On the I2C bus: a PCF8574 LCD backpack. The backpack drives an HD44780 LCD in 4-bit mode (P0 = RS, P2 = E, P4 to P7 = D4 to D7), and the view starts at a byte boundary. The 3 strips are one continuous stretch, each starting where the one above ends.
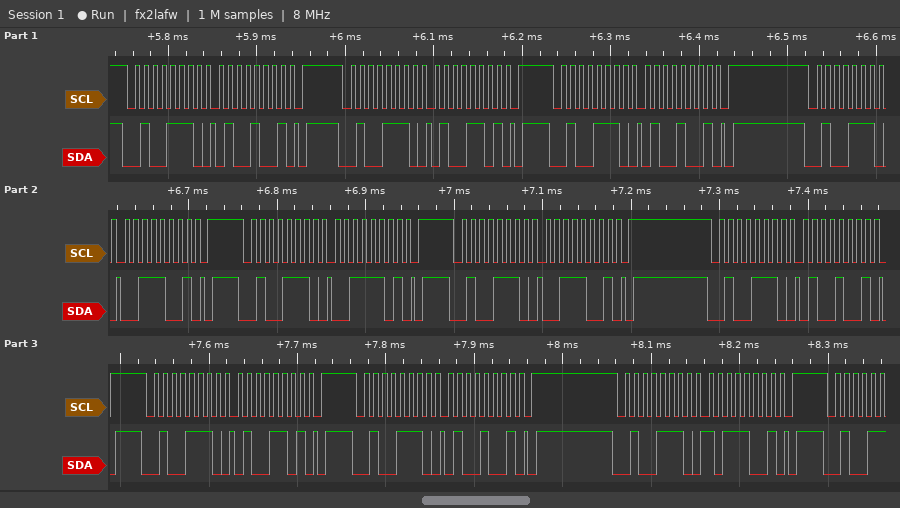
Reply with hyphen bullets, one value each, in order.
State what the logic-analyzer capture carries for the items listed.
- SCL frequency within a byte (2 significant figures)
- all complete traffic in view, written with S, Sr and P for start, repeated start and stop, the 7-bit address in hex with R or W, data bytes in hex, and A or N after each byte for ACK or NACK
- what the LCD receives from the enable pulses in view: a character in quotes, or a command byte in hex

- 100 kHz
- S 27W A 49 A P S 27W A 4D A P S 27W A 49 A P S 27W A 39 A P S 27W A 3D A P S 27W A 39 A P S 27W A 49 A P S 27W A 4D A P S 27W A 49 A P S 27W A B9 A P
- 'C'
